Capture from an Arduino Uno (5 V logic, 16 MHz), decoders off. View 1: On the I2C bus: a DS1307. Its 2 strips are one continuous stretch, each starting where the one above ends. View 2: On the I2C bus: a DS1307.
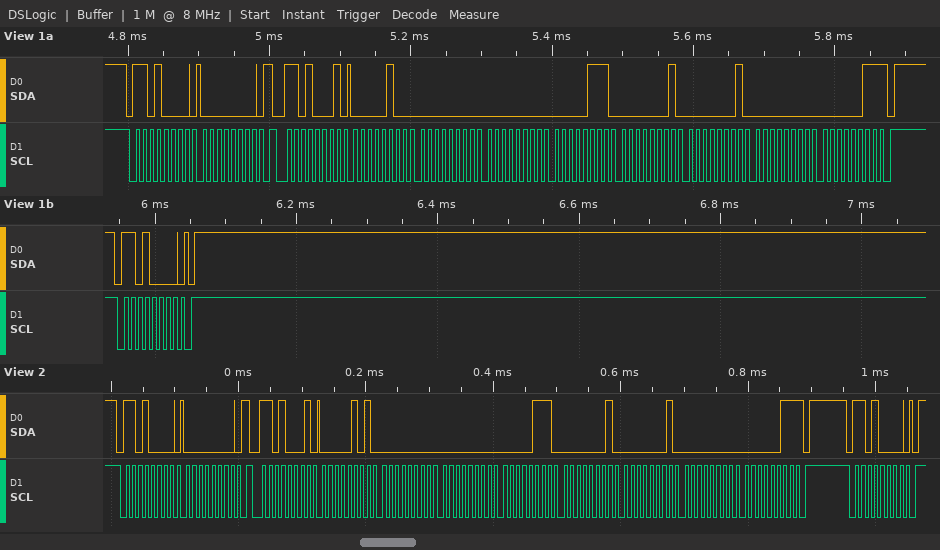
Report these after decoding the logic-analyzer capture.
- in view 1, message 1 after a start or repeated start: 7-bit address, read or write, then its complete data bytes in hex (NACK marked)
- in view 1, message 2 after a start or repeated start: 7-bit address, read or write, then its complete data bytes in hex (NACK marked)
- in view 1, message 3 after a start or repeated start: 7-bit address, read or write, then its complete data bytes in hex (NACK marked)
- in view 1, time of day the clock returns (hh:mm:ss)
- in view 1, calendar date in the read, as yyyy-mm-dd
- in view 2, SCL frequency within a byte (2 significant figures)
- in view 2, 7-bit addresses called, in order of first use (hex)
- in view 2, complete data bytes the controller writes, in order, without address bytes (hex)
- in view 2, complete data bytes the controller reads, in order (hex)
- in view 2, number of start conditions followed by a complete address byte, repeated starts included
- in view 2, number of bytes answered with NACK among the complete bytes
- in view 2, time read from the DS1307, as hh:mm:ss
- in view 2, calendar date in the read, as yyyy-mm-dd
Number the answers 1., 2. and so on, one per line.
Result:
1. 0x68 write: 00
2. 0x68 read: 04 00 00 07 01 01 00 03 NACK
3. 0x68 write
4. 00:00:04
5. 2000-01-01
6. 100 kHz
7. 0x68
8. 00
9. 05 00 00 07 01 01 00 03
10. 3
11. 1
12. 00:00:05
13. 2000-01-01
